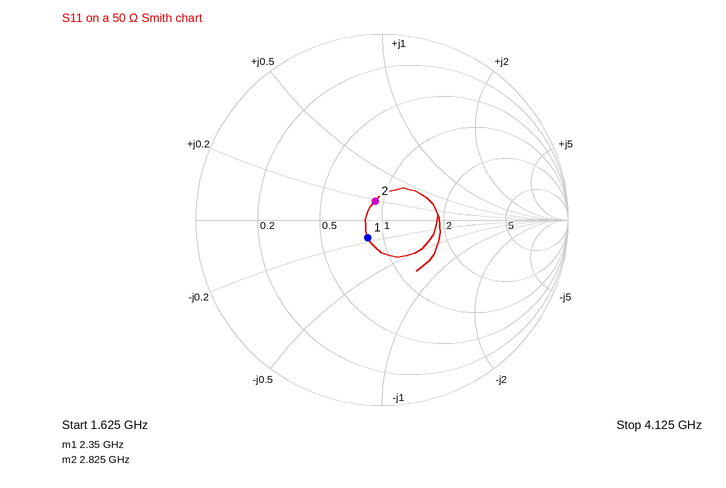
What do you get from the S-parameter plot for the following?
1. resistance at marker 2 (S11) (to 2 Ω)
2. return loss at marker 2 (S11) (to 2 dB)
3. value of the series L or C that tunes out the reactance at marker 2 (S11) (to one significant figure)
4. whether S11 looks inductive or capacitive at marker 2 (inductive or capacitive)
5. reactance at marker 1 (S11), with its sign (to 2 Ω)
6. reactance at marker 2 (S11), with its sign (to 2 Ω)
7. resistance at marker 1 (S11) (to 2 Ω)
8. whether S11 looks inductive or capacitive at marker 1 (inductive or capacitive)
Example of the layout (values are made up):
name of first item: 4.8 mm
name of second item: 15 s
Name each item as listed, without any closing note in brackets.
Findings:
resistance at marker 2 (S11): 46 Ω
return loss at marker 2 (S11): 20 dB
value of the series L or C that tunes out the reactance at marker 2 (S11): 6 pF
whether S11 looks inductive or capacitive at marker 2: inductive
reactance at marker 1 (S11), with its sign: -8 Ω
reactance at marker 2 (S11), with its sign: +10 Ω
resistance at marker 1 (S11): 42 Ω
whether S11 looks inductive or capacitive at marker 1: capacitive
